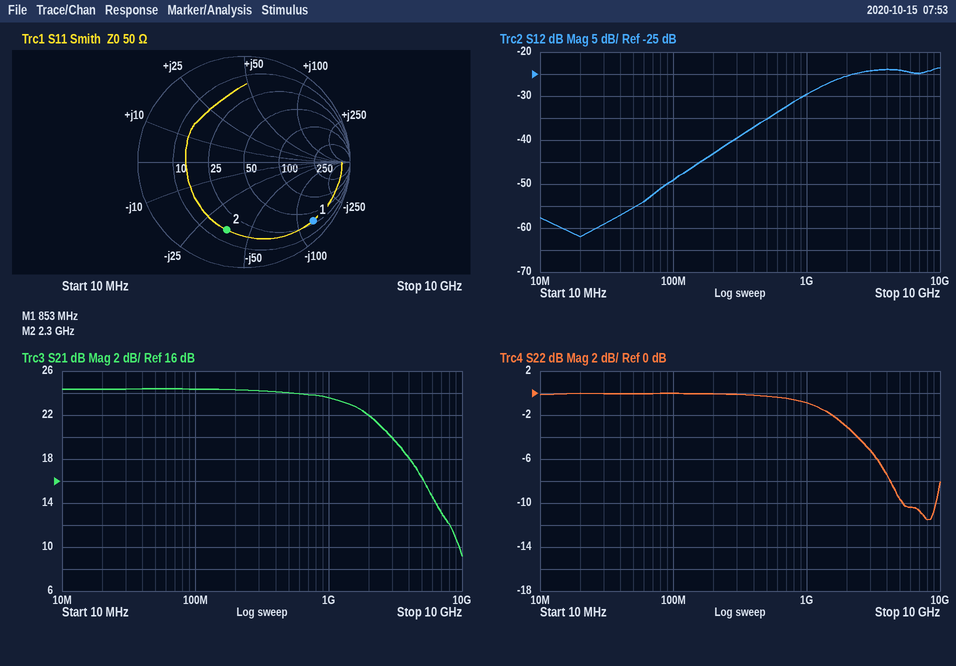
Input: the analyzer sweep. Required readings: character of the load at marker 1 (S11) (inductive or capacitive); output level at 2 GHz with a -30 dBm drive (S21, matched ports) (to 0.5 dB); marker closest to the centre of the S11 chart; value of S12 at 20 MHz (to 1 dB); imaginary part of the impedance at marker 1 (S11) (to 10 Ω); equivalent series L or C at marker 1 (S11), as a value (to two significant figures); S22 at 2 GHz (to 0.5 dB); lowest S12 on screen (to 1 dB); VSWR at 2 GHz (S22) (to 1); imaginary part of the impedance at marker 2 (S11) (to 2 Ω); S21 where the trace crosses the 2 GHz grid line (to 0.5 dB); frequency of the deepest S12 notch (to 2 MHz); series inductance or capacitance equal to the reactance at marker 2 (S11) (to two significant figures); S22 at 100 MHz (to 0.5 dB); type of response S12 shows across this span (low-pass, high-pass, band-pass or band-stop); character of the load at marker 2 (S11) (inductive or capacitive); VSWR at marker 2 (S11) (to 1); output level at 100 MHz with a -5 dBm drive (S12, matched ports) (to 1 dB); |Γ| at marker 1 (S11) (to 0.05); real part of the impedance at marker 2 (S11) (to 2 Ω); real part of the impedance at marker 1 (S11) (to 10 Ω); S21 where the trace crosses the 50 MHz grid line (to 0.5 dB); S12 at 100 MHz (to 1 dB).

capacitive
-8.0 dBm
marker 2
-62 dB
-130 Ω
1.4 pF
-3.0 dB
-62 dB
6
-36 Ω
22.0 dB
20 MHz
1.9 pF
0.0 dB
high-pass
capacitive
5
-54 dBm
0.85
16 Ω
30 Ω
24.5 dB
-49 dB
